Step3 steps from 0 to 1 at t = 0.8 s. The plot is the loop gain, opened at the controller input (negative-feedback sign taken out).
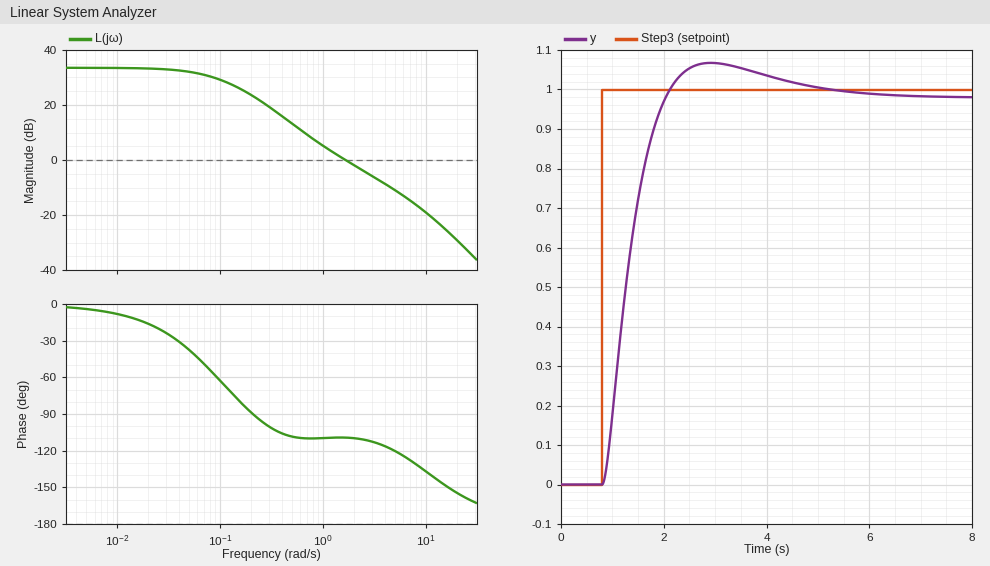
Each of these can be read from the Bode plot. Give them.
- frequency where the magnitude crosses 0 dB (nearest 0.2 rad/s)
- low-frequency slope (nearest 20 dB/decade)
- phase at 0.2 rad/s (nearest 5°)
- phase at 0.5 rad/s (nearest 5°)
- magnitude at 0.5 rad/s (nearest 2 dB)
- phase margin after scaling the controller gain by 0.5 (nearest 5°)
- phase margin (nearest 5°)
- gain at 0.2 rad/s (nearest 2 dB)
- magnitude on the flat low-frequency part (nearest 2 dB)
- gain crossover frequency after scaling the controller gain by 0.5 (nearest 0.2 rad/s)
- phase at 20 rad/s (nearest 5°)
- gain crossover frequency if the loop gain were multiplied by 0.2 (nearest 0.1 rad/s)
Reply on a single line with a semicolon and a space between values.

1.6 rad/s; 0 dB/decade; -90°; -110°; 14 dB; 70°; 70°; 24 dB; 34 dB; 1.0 rad/s; -155°; 0.5 rad/s
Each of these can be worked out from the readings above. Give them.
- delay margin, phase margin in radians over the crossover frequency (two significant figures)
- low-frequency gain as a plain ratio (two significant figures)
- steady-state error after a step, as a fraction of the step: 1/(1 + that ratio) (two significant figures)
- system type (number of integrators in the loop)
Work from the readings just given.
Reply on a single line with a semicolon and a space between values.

0.76 s; 50; 0.020; 0
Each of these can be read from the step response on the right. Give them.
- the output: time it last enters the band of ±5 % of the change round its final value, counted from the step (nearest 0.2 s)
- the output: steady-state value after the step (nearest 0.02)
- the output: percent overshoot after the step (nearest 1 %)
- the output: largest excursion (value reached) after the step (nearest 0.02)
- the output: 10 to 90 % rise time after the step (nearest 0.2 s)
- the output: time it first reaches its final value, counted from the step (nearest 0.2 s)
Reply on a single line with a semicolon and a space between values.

3.4 s; 0.98; 9 %; 1.06; 0.8 s; 1.2 s
